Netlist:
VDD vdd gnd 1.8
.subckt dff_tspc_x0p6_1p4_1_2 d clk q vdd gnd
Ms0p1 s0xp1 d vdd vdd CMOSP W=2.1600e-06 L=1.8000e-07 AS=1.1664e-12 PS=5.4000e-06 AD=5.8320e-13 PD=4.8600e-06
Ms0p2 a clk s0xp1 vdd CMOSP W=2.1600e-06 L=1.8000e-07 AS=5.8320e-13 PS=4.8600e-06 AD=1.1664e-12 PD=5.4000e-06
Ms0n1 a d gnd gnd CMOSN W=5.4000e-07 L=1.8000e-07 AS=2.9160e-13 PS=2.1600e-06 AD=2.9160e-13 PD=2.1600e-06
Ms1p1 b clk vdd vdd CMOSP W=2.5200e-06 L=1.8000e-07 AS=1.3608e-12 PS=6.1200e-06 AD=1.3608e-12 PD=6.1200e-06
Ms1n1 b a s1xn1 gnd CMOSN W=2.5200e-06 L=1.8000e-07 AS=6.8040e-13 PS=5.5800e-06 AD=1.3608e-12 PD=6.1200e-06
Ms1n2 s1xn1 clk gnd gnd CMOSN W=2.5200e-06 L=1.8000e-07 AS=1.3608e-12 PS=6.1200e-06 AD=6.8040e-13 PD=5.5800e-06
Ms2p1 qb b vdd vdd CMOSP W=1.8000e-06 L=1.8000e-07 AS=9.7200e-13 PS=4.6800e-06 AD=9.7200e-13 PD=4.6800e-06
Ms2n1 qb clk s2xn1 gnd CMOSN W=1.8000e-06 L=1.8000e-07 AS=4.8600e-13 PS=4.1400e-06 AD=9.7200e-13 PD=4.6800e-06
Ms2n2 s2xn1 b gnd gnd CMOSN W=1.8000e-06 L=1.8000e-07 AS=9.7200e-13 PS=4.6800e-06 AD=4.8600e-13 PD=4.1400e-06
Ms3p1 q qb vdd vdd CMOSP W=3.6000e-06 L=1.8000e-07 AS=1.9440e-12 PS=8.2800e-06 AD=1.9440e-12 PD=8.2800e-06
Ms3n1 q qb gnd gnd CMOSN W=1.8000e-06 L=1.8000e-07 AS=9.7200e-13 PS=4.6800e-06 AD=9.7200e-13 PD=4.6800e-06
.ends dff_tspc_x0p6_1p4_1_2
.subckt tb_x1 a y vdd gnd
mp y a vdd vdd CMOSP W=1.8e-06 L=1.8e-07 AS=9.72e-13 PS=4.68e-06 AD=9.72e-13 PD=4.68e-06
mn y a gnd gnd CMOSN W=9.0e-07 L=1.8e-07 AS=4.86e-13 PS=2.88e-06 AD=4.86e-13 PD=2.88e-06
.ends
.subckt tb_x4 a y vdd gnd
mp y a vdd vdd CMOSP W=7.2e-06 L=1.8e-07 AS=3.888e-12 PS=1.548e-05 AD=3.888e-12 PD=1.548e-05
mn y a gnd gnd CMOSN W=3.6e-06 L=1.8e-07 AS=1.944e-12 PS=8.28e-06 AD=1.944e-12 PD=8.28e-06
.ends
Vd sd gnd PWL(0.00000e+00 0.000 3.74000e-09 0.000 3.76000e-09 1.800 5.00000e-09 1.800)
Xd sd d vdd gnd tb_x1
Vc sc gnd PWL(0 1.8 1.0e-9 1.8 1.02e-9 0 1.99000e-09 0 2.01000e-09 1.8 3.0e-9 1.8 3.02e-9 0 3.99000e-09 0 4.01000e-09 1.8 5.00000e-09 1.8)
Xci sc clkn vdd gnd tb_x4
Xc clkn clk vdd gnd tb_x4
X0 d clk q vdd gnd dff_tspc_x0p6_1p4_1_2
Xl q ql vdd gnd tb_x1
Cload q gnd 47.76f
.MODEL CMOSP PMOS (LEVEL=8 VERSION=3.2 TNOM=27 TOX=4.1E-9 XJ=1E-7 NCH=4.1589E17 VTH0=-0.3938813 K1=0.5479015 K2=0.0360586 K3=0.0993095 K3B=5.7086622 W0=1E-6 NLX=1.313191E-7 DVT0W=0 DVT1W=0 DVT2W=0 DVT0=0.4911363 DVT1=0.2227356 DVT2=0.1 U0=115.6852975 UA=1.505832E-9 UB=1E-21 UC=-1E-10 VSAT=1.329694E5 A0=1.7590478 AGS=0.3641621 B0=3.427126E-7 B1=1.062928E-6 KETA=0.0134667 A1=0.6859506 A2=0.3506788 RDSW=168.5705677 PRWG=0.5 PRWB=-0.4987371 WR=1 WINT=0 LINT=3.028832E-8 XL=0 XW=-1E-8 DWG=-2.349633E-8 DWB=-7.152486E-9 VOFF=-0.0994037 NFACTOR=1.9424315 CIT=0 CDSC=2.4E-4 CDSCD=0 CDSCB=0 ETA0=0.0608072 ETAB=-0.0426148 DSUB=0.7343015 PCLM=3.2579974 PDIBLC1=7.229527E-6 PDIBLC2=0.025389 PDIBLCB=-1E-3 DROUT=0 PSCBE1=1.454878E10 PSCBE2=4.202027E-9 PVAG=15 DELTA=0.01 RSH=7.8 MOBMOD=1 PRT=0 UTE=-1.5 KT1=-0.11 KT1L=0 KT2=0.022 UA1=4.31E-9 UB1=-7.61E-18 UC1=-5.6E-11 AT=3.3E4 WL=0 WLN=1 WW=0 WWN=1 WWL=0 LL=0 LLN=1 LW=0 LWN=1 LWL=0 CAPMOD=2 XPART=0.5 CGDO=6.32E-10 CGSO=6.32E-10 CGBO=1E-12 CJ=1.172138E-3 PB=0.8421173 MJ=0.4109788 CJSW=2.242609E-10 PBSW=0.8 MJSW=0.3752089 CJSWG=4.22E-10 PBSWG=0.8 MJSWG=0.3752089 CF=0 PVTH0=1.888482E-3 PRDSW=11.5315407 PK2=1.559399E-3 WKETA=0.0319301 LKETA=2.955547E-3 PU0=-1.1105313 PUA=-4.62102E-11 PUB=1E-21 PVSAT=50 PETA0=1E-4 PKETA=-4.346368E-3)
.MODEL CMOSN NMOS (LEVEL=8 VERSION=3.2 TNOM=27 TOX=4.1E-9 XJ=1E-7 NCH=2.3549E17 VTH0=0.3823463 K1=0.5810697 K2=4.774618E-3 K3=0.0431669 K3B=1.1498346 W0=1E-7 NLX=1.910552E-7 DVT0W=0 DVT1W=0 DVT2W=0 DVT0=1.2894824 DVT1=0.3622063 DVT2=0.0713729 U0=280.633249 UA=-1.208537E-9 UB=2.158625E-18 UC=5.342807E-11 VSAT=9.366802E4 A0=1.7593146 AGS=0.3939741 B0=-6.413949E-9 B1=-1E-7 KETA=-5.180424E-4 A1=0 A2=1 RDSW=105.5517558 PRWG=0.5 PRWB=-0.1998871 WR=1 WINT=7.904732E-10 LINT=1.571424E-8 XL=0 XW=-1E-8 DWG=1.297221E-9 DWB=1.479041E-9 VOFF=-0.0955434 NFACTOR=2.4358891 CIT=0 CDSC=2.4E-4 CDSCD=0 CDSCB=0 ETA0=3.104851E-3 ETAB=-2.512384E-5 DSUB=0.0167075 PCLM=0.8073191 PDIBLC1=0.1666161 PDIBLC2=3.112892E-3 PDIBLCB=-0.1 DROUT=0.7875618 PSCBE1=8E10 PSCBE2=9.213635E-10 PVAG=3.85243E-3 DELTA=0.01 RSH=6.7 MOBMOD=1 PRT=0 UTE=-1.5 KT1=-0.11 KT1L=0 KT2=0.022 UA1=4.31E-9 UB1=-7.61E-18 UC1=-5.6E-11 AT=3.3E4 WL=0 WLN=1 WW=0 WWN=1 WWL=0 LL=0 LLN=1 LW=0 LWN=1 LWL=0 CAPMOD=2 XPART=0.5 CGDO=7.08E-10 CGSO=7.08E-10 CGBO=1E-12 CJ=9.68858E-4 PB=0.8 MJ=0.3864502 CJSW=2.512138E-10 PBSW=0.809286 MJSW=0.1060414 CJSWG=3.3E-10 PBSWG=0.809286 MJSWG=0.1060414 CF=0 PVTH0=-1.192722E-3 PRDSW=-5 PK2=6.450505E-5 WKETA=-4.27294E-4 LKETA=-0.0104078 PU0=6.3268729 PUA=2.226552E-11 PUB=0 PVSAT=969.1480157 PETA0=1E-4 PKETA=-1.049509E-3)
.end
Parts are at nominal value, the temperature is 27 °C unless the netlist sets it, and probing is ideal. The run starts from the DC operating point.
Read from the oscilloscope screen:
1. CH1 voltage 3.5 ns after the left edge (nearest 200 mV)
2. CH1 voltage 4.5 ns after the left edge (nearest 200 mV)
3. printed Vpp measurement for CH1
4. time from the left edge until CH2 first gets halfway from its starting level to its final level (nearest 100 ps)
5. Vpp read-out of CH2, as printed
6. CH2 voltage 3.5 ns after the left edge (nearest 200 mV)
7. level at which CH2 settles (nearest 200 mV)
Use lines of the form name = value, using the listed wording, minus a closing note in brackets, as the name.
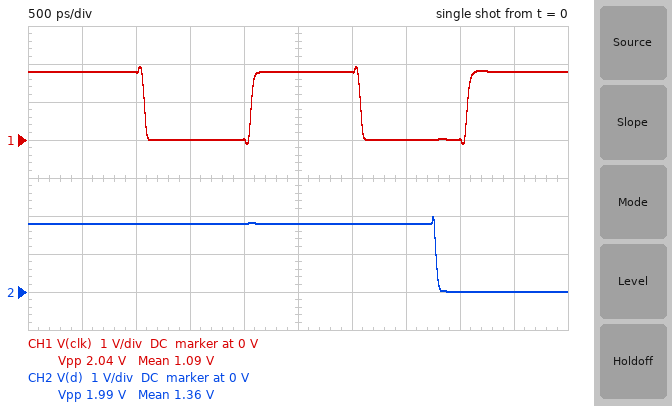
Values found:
CH1 voltage 3.5 ns after the left edge = 0 V
CH1 voltage 4.5 ns after the left edge = 1.8 V
printed Vpp measurement for CH1 = 2.04 V
time from the left edge until CH2 first gets halfway from its starting level to its final level = 3.8 ns
Vpp read-out of CH2, as printed = 1.99 V
CH2 voltage 3.5 ns after the left edge = 1.8 V
level at which CH2 settles = 0 V
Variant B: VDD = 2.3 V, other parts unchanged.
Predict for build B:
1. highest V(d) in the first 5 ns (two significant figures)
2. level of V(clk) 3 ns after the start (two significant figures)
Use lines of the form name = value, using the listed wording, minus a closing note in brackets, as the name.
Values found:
highest V(d) in the first 5 ns = 2.5 V
level of V(clk) 3 ns after the start = 2.3 V
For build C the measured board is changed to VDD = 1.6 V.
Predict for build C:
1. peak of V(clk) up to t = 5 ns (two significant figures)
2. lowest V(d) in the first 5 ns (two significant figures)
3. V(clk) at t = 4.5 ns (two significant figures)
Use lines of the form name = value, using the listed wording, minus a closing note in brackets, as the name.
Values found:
peak of V(clk) up to t = 5 ns = 1.7 V
lowest V(d) in the first 5 ns = -8.7 mV
V(clk) at t = 4.5 ns = 1.6 V
